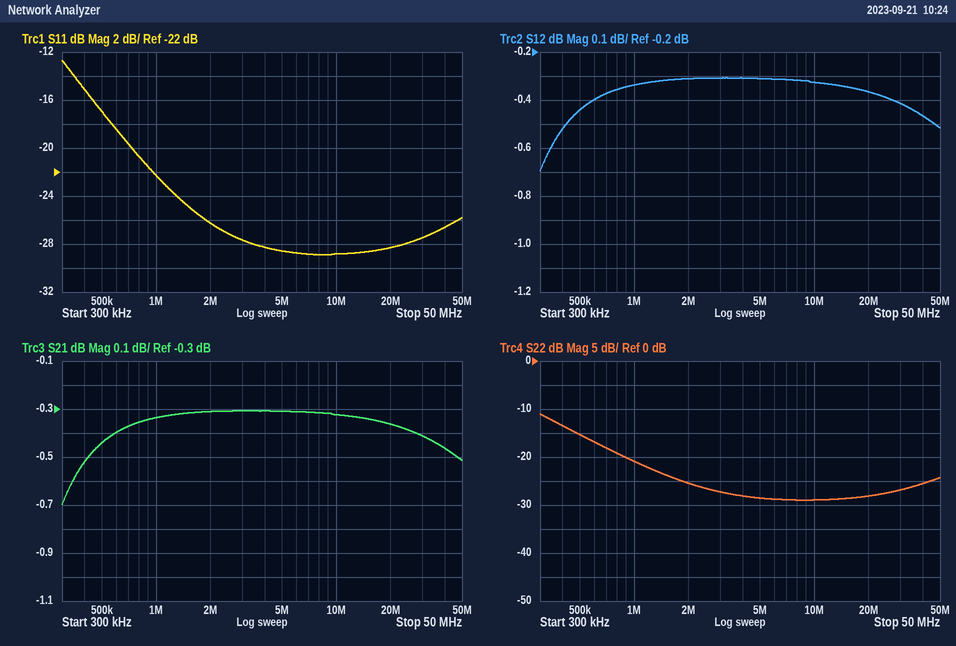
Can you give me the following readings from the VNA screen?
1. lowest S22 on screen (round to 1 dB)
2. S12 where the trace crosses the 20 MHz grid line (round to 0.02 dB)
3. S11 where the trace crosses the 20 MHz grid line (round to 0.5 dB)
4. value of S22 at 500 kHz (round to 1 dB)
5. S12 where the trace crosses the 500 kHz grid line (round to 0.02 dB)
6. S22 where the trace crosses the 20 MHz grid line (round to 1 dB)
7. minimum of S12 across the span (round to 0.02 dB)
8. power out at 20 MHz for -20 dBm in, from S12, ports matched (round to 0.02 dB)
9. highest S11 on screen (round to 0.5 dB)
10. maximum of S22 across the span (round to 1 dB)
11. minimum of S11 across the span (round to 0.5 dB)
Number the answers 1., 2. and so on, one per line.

1. -29 dB
2. -0.36 dB
3. -28.5 dB
4. -15 dB
5. -0.44 dB
6. -28 dB
7. -0.70 dB
8. -20.36 dBm
9. -12.5 dB
10. -11 dB
11. -29.0 dB
